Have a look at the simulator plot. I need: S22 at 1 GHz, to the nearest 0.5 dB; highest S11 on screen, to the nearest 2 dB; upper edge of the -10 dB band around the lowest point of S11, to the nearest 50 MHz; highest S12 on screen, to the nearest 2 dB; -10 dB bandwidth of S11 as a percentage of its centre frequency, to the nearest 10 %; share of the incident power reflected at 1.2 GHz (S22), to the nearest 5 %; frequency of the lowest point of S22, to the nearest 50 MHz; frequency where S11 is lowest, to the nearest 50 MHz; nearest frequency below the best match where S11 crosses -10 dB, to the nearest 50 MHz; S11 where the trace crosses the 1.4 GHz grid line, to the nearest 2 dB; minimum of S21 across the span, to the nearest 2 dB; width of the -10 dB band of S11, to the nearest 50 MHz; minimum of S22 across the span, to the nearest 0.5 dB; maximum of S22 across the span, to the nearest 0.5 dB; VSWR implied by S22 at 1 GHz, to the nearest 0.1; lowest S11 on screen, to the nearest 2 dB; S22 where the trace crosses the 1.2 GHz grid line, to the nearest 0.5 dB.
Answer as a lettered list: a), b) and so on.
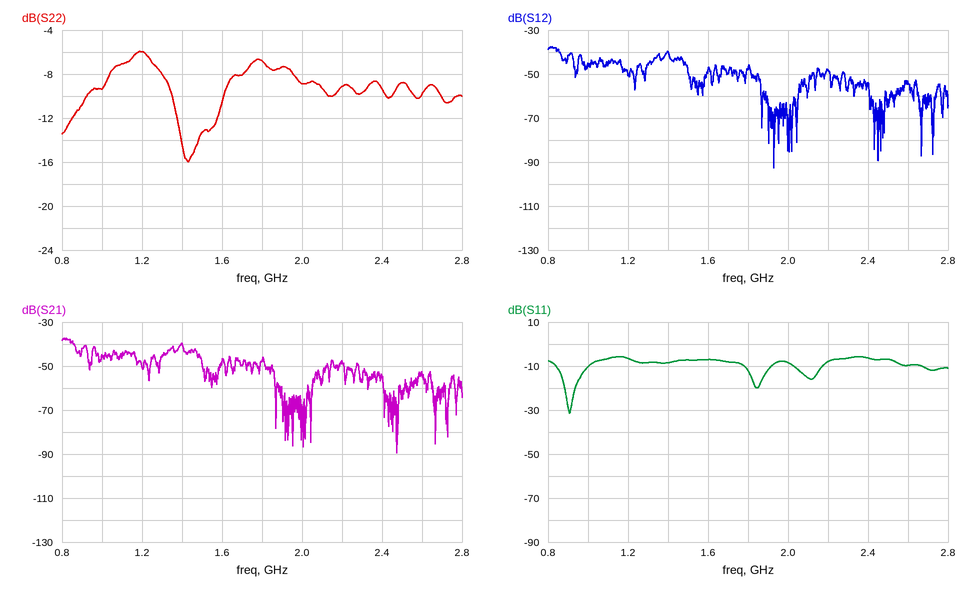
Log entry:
a) -9.5 dB
b) -6 dB
c) 1.00 GHz
d) -38 dB
e) 20 %
f) 25 %
g) 1.45 GHz
h) 900 MHz
i) 850 MHz
j) -8 dB
k) -90 dB
l) 150 MHz
m) -16.0 dB
n) -6.0 dB
o) 2.0
p) -32 dB
q) -6.0 dB
